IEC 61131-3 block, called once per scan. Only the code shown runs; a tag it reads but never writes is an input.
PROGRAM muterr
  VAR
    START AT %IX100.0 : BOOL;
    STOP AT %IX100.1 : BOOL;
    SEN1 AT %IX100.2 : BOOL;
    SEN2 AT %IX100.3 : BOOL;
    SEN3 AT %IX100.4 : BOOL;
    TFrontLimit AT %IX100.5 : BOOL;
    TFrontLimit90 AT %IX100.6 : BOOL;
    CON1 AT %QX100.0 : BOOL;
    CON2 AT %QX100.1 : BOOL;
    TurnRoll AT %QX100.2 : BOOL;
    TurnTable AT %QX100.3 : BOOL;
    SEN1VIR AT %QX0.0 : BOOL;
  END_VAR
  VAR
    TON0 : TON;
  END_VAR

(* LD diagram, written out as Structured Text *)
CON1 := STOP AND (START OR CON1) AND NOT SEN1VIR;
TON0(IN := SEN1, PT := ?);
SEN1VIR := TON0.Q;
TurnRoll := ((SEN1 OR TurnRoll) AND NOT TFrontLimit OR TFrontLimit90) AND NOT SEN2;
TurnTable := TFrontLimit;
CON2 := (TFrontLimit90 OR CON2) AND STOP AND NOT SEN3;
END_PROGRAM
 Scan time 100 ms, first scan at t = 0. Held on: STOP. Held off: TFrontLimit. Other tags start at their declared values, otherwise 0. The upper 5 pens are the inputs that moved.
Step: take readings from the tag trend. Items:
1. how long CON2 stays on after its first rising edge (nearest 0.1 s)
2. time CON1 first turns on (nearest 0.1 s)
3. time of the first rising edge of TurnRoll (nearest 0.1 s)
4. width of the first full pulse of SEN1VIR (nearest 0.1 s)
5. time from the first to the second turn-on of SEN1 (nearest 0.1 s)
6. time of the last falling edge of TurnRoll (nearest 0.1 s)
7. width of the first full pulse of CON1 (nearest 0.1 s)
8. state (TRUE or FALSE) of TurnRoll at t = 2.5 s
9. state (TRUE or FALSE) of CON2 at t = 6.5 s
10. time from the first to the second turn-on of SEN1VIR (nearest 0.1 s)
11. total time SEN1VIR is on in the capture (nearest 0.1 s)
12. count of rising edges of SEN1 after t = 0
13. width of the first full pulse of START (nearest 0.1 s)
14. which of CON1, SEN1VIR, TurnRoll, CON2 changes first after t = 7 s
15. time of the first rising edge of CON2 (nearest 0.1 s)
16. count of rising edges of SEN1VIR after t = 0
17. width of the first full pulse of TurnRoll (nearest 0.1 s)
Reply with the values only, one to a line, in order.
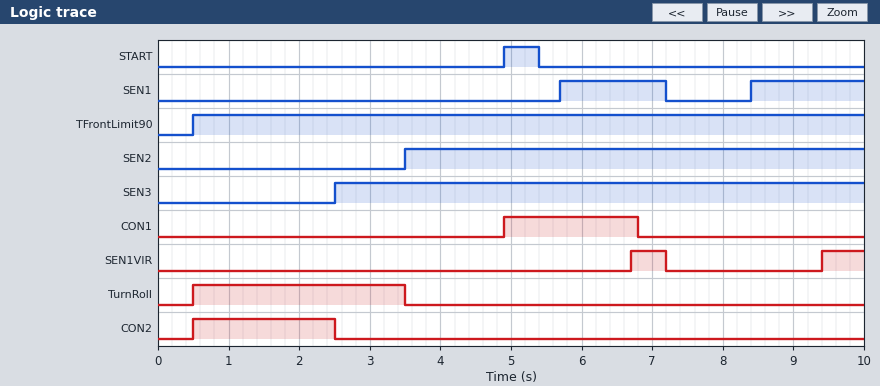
2.0 s
4.9 s
0.5 s
0.5 s
2.7 s
3.5 s
1.9 s
TRUE
FALSE
2.7 s
1.1 s
2
0.5 s
SEN1VIR
0.5 s
2
3.0 s
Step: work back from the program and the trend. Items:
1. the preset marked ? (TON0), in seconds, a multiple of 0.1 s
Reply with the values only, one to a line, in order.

1.0 s
